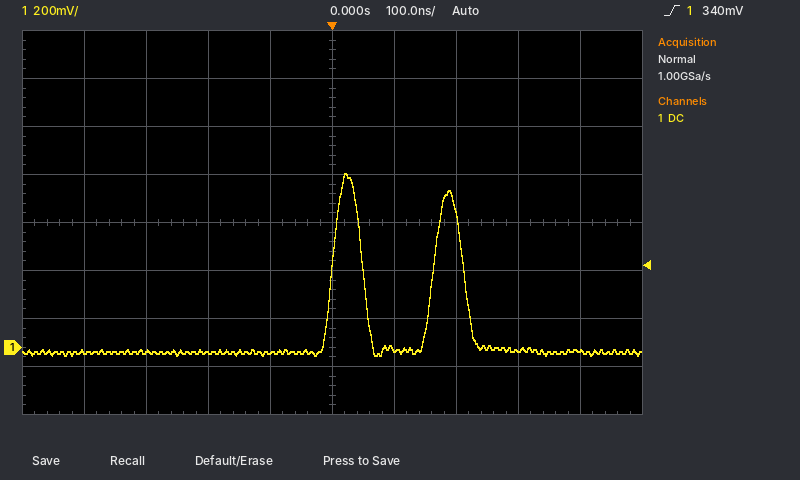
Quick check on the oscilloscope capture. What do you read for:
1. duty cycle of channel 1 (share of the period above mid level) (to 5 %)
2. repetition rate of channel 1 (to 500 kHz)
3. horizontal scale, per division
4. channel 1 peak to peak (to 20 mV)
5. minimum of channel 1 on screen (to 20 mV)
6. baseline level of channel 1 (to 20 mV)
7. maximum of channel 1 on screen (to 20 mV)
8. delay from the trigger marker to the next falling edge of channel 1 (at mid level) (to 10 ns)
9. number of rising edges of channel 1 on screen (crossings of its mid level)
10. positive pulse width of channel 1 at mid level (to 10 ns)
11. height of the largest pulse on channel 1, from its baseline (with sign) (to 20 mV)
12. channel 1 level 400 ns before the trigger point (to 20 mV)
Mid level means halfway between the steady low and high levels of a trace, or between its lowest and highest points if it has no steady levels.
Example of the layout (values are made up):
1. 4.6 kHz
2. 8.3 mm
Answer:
1. 30 %
2. 6.0 MHz
3. 100 ns
4. 760 mV
5. -40 mV
6. -20 mV
7. 720 mV
8. 50 ns
9. 2
10. 50 ns
11. +740 mV
12. -20 mV
